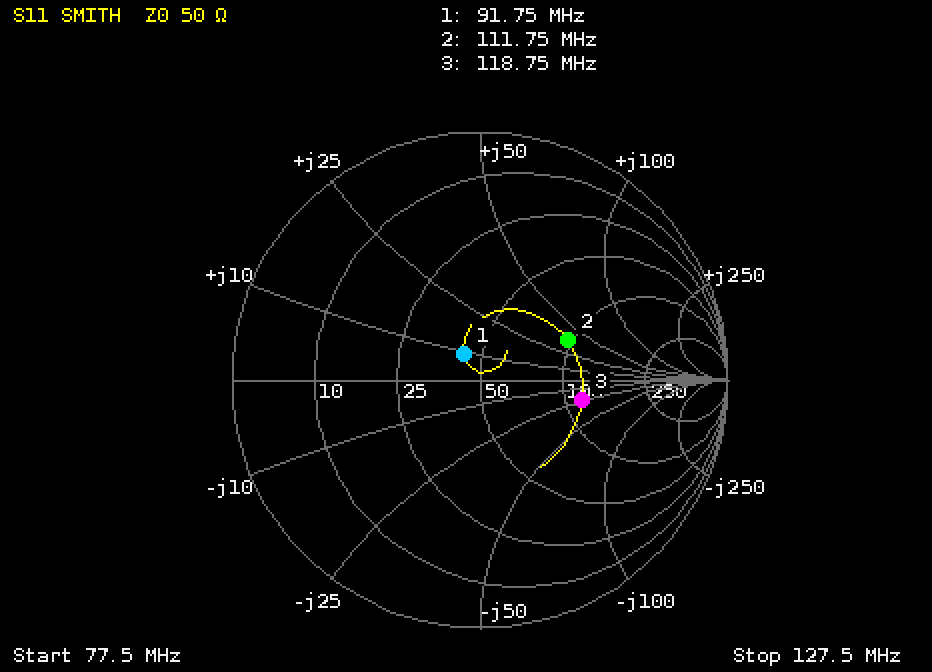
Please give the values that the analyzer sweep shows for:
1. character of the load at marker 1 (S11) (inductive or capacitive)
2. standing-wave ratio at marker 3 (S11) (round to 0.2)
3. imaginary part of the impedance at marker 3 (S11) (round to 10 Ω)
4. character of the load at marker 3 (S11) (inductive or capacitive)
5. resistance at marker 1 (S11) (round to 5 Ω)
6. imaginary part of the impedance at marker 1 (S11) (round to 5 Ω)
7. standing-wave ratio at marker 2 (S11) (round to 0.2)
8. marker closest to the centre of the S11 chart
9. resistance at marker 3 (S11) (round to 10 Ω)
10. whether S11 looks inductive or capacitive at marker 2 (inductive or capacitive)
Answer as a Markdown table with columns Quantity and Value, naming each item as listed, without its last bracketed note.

| Quantity | Value |
|---|---|
| character of the load at marker 1 (S11) | inductive |
| standing-wave ratio at marker 3 (S11) | 2.4 |
| imaginary part of the impedance at marker 3 (S11) | -20 Ω |
| character of the load at marker 3 (S11) | capacitive |
| resistance at marker 1 (S11) | 45 Ω |
| imaginary part of the impedance at marker 1 (S11) | +10 Ω |
| standing-wave ratio at marker 2 (S11) | 2.2 |
| marker closest to the centre of the S11 chart | marker 1 |
| resistance at marker 3 (S11) | 120 Ω |
| whether S11 looks inductive or capacitive at marker 2 | inductive |
